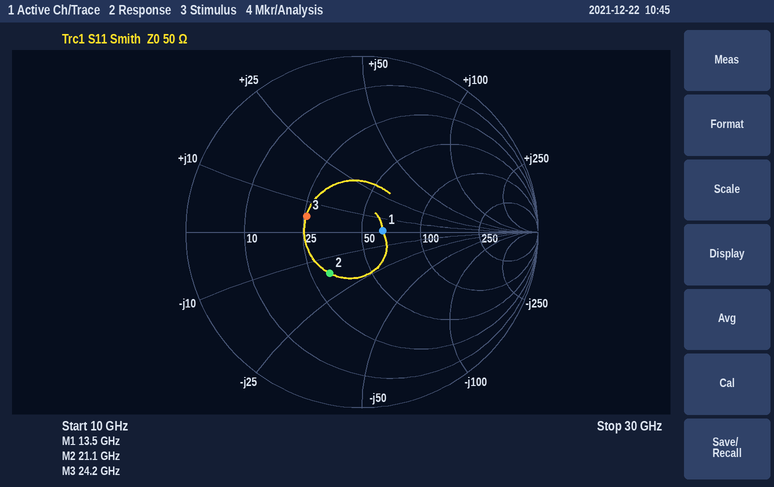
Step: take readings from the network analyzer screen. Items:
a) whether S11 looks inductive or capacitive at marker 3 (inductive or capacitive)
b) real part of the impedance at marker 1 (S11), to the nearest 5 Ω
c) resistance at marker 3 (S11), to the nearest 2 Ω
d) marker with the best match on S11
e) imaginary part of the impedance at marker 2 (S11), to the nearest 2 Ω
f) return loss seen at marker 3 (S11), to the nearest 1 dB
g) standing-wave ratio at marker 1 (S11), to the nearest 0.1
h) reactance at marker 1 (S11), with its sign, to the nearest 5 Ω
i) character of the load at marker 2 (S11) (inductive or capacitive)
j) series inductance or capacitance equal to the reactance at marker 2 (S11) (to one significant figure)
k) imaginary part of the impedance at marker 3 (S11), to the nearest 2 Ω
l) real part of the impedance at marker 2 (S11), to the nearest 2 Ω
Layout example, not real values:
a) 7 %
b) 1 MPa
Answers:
a) inductive
b) 65 Ω
c) 26 Ω
d) marker 1
e) -16 Ω
f) 10 dB
g) 1.3
h) 0 Ω
i) capacitive
j) 500 fF
k) +6 Ω
l) 32 Ω
